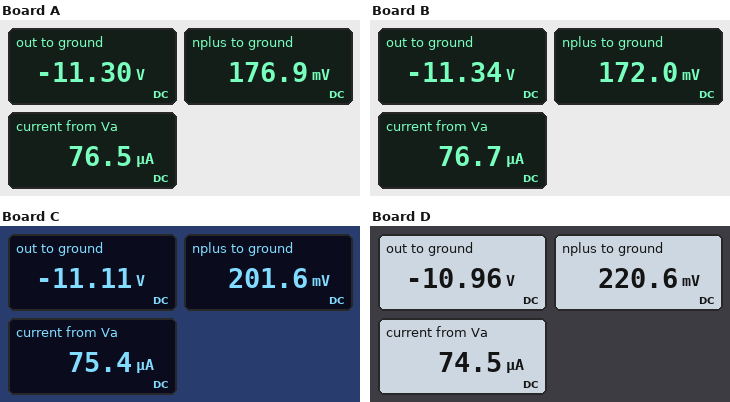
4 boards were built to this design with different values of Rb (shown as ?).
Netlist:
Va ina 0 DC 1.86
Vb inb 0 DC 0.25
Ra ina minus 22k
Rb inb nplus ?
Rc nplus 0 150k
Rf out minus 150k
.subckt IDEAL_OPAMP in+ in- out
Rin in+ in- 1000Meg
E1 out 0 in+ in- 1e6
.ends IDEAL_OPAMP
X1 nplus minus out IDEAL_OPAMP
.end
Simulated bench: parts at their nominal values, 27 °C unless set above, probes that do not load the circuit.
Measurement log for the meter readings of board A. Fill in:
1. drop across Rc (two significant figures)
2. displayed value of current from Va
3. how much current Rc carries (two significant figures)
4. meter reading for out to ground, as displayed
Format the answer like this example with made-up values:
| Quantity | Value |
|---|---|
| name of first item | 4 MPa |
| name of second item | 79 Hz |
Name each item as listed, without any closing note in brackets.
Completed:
| Quantity | Value |
|---|---|
| drop across Rc | 180 mV |
| displayed value of current from Va | 76.5 µA |
| how much current Rc carries | 1.2 µA |
| meter reading for out to ground, as displayed | -11.30 V |
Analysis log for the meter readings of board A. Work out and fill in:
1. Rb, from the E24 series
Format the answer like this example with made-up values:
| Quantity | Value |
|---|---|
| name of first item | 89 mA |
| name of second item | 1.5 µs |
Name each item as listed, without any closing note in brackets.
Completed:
| Quantity | Value |
|---|---|
| Rb, from the E24 series | 62 kΩ |
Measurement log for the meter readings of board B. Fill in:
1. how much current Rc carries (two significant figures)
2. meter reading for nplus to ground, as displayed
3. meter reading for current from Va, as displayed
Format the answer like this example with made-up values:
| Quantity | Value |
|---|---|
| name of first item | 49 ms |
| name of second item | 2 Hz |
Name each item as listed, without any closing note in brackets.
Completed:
| Quantity | Value |
|---|---|
| how much current Rc carries | 1.1 µA |
| meter reading for nplus to ground, as displayed | 172.0 mV |
| meter reading for current from Va, as displayed | 76.7 µA |
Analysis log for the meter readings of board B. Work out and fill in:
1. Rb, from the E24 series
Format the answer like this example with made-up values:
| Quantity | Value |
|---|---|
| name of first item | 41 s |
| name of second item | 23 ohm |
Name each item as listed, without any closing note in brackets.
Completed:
| Quantity | Value |
|---|---|
| Rb, from the E24 series | 68 kΩ |
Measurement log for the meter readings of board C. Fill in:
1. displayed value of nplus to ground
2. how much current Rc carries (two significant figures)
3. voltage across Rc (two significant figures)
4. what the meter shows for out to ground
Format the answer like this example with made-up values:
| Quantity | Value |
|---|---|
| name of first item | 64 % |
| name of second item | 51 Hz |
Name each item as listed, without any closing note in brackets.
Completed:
| Quantity | Value |
|---|---|
| displayed value of nplus to ground | 201.6 mV |
| how much current Rc carries | 1.3 µA |
| voltage across Rc | 200 mV |
| what the meter shows for out to ground | -11.11 V |
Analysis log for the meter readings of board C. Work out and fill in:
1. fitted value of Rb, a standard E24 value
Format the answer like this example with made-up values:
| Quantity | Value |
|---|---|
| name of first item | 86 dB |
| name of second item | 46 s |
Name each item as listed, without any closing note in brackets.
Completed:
| Quantity | Value |
|---|---|
| fitted value of Rb, a standard E24 value | 36 kΩ |
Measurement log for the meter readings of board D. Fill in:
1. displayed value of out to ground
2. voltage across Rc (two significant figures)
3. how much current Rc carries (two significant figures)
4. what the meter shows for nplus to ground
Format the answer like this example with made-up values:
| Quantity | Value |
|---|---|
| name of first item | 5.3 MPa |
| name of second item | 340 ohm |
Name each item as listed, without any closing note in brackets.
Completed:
| Quantity | Value |
|---|---|
| displayed value of out to ground | -10.96 V |
| voltage across Rc | 220 mV |
| how much current Rc carries | 1.5 µA |
| what the meter shows for nplus to ground | 220.6 mV |
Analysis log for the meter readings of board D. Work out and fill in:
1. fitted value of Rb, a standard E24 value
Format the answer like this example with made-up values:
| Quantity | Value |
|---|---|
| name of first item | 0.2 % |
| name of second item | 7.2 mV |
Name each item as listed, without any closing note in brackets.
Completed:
| Quantity | Value |
|---|---|
| fitted value of Rb, a standard E24 value | 20 kΩ |
